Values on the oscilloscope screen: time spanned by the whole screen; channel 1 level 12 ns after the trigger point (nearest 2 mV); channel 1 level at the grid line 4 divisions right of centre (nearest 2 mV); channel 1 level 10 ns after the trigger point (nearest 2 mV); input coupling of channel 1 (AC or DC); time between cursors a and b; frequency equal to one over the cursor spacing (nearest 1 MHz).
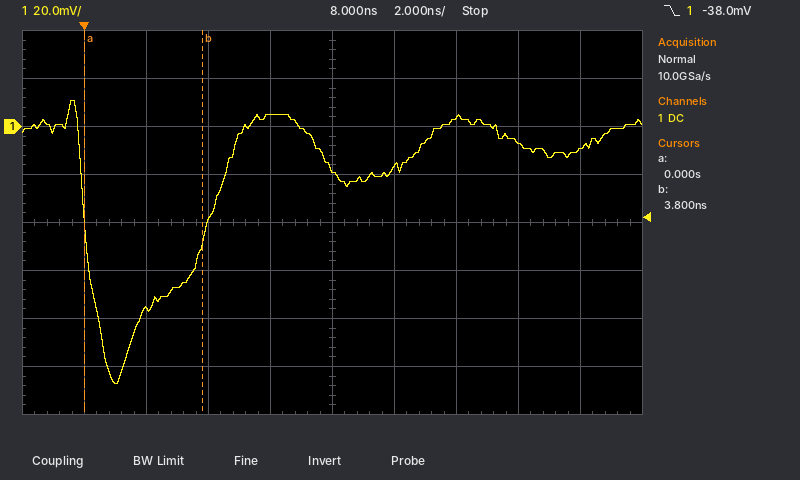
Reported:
20 ns
4 mV
-10 mV
-16 mV
DC
3.8 ns
263 MHz
